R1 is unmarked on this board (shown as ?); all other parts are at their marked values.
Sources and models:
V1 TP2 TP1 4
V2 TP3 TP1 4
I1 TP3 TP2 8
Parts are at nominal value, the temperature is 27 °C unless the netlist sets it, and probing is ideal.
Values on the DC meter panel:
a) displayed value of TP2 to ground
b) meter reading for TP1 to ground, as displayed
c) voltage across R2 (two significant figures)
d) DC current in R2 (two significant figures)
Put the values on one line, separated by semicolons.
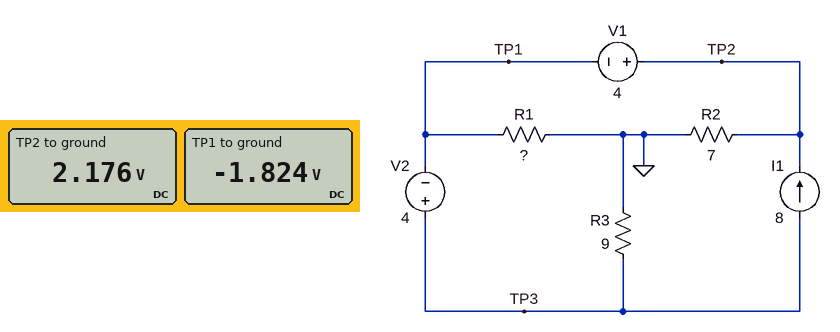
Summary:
2.176 V; -1.824 V; 2.2 V; 310 mA
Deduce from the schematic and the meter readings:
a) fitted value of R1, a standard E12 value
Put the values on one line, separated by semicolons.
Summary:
3.3 Ω
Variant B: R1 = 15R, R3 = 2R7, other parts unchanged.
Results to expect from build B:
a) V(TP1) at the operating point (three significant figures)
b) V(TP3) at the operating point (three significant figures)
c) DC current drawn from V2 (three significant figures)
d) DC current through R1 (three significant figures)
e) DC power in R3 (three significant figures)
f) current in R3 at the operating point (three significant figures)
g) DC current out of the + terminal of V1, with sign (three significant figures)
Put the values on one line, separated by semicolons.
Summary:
-3.54 V; 460 mV; 8.17 A; 236 mA; 78.3 mW; 170 mA; -7.93 A
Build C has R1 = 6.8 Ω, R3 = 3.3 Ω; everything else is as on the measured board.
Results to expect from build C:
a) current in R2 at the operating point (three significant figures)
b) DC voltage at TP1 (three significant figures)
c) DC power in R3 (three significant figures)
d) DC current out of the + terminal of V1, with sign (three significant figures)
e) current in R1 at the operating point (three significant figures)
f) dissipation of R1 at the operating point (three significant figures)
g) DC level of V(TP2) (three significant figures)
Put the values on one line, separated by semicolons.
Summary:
142 mA; -3.01 V; 298 mW; -7.86 A; 442 mA; 1.33 W; 992 mV
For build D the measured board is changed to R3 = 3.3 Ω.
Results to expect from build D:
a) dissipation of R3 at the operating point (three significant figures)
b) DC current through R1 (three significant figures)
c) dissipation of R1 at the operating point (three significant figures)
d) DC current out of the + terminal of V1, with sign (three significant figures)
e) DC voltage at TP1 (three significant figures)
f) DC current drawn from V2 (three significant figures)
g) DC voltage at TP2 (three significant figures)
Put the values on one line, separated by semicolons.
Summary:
794 mW; 722 mA; 1.72 W; -7.77 A; -2.38 V; 8.49 A; 1.62 V
